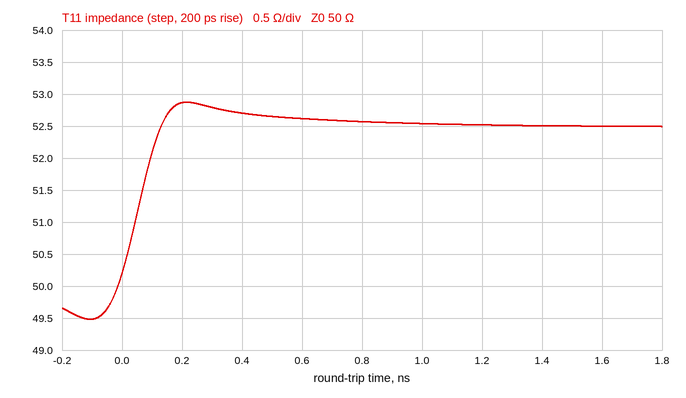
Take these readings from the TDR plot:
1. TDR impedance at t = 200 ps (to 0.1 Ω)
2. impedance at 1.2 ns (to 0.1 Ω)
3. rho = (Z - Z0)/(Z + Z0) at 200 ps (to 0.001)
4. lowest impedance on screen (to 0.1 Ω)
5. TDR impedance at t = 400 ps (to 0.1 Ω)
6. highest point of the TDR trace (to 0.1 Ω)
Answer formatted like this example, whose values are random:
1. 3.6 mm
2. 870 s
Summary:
1. 52.9 Ω
2. 52.5 Ω
3. +0.028
4. 49.5 Ω
5. 52.7 Ω
6. 52.9 Ω
